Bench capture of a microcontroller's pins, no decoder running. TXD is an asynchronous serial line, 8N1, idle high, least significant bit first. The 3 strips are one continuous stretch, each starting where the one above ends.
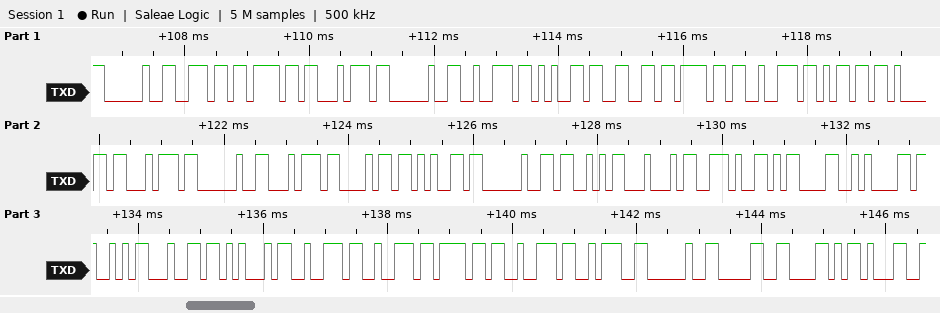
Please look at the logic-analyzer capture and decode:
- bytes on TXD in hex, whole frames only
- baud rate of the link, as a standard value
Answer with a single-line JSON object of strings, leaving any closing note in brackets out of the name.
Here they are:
{"bytes on TXD in hex, whole frames only": "20 6E 6F 74 20 72 65 66 6F 72 6D 61 74 20 74 68 65 20 53 44 2E 0D 0A 53 64 45 72 72 6F 72 3A 20 30 58 31", "baud rate of the link, as a standard value": "9600 baud"}
